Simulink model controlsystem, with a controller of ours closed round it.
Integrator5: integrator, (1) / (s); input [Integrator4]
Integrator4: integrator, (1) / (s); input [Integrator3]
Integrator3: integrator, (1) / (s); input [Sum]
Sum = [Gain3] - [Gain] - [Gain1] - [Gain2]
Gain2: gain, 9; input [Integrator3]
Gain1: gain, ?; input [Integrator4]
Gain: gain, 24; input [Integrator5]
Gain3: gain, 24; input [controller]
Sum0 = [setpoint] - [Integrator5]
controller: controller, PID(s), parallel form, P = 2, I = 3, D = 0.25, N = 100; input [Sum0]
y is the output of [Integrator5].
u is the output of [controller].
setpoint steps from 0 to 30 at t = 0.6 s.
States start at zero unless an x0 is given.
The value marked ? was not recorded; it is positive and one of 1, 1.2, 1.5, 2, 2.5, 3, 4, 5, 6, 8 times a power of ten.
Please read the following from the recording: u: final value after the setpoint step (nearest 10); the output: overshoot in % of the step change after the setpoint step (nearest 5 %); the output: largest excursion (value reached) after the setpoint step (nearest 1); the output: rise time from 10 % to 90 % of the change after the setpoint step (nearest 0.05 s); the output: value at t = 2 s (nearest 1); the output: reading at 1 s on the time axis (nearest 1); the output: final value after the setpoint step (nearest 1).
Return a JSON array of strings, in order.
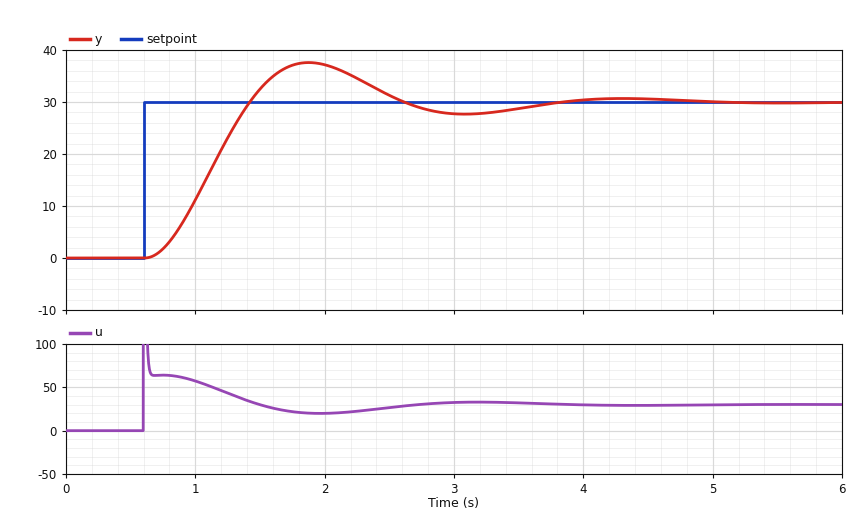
["30", "25 %", "38", "0.55 s", "37", "11", "30"]
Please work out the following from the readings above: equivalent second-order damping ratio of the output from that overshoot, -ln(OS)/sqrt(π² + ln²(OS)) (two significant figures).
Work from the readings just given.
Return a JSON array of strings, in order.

["0.40"]
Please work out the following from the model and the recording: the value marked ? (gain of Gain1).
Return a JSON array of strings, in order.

["25"]
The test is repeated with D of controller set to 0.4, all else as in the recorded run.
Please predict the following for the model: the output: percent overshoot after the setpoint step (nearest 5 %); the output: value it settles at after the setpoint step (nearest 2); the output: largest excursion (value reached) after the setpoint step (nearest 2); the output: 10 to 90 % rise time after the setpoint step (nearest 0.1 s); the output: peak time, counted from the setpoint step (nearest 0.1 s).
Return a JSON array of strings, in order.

["15 %", "30", "34", "0.6 s", "1.3 s"]
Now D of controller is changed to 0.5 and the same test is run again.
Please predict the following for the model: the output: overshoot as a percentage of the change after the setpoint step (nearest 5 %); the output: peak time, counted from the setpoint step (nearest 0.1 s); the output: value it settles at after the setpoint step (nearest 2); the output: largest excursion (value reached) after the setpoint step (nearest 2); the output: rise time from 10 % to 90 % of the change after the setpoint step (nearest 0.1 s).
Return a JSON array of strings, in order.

["10 %", "1.3 s", "30", "34", "0.6 s"]
